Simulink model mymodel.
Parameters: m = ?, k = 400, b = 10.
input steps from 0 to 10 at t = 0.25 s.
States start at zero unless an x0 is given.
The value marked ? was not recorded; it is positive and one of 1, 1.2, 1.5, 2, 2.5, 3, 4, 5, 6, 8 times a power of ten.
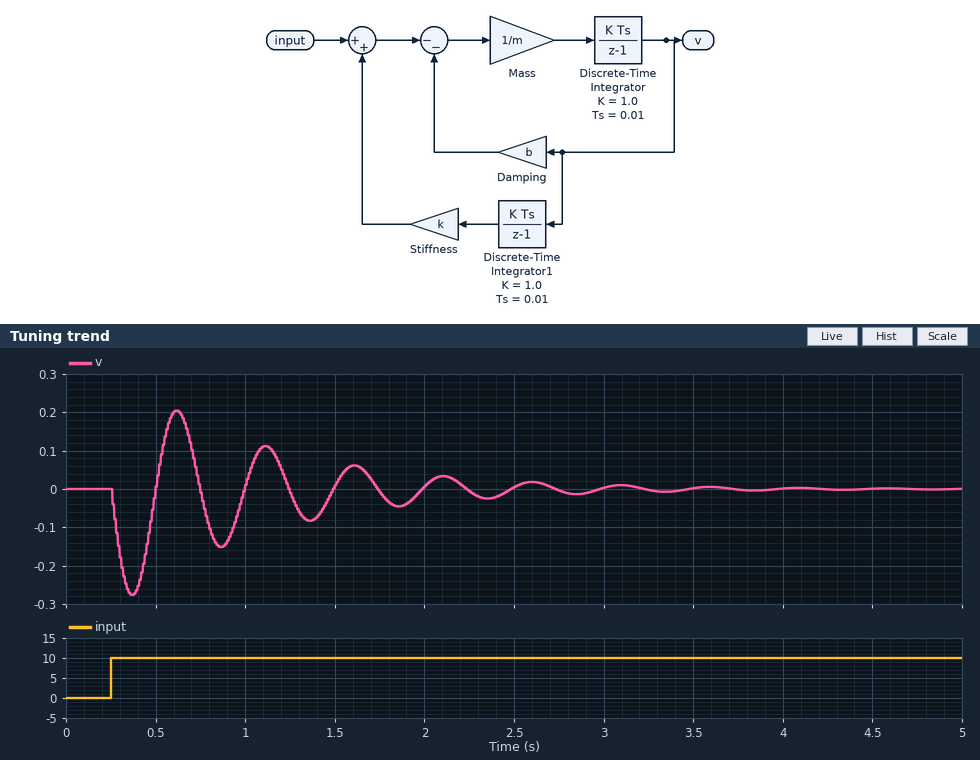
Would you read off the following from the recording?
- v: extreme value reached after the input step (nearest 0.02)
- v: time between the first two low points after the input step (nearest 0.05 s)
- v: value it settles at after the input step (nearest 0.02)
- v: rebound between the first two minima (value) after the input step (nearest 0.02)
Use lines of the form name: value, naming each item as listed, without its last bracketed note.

v: extreme value reached after the input step: -0.28
v: time between the first two low points after the input step: 0.50 s
v: value it settles at after the input step: 0.00
v: rebound between the first two minima (value) after the input step: 0.20
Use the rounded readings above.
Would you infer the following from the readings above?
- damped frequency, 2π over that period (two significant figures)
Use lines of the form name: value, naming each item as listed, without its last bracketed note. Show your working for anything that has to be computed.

damped frequency, 2π over that period: 2π / 0.5 = 13 rad/s
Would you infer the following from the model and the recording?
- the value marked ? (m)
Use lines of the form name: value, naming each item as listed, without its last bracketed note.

the value marked ?: 2.5
